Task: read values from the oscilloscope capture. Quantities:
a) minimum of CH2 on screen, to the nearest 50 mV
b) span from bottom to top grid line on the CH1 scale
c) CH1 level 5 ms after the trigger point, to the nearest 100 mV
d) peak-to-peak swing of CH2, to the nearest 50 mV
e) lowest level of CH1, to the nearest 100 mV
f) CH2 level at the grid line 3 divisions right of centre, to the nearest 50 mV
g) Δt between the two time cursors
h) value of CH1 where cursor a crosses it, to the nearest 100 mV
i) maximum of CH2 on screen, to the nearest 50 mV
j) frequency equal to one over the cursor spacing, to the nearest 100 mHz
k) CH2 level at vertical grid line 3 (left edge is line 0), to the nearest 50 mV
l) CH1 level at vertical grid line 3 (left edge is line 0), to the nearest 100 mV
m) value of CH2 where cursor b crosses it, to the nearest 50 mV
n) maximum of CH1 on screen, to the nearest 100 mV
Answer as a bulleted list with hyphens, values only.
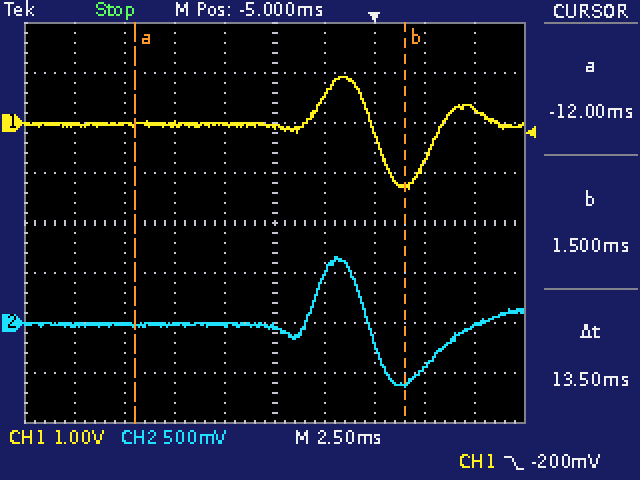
- -650 mV
- 8 V
- 300 mV
- 1.30 V
- -1.3 V
- -450 mV
- 13.5 ms
- 0.0 V
- 650 mV
- 74.1 Hz
- 0 mV
- 0.0 V
- -600 mV
- 900 mV
